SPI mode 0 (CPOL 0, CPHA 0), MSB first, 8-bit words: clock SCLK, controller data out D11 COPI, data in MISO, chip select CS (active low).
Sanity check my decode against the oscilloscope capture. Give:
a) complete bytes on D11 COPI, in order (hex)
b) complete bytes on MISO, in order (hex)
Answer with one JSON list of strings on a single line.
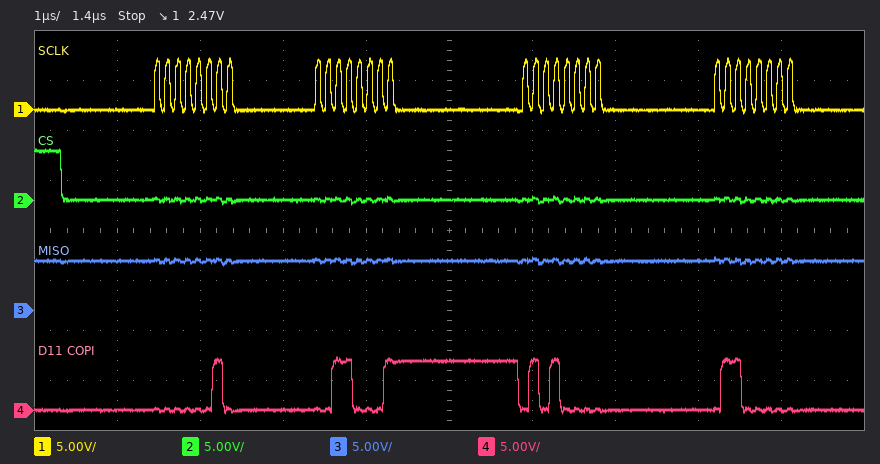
["02 31 50 60", "FF FF FF FF"]
